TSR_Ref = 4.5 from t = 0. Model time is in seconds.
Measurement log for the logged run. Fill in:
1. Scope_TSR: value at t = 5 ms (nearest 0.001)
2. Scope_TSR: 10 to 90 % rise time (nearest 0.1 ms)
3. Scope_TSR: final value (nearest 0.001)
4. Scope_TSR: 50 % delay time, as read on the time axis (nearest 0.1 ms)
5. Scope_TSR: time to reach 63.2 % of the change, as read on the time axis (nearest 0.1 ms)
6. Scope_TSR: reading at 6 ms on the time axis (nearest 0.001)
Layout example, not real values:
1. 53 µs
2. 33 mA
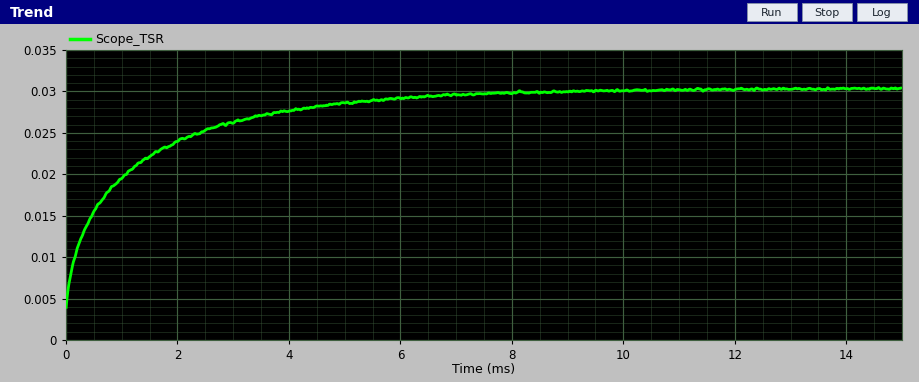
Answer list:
1. 0.029
2. 4.0 ms
3. 0.030
4. 0.7 ms
5. 1.2 ms
6. 0.029
